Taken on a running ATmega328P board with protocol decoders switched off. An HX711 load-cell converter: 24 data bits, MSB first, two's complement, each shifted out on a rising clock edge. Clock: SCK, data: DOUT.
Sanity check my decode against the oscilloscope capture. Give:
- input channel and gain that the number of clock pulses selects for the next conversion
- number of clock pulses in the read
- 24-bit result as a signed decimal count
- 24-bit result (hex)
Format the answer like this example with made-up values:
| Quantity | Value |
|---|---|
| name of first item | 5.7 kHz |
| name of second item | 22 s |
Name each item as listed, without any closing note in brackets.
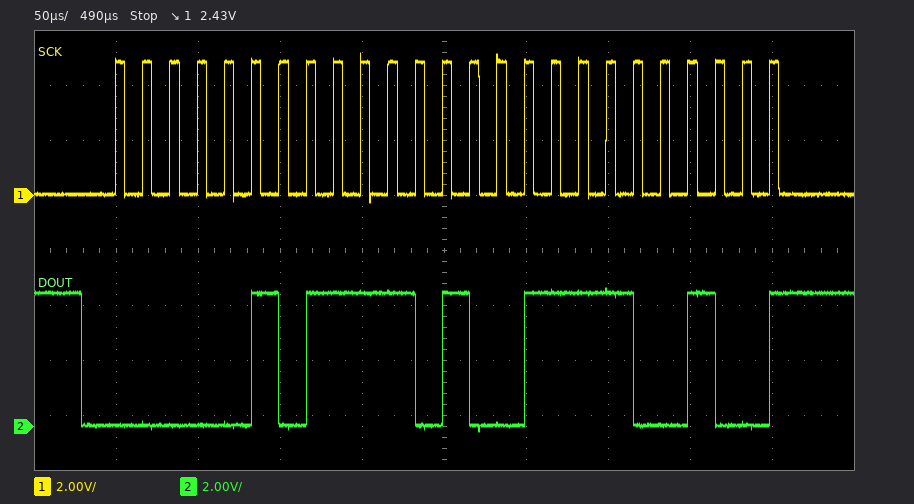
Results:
| Quantity | Value |
|---|---|
| input channel and gain that the number of clock pulses selects for the next conversion | channel A, gain 128 |
| number of clock pulses in the read | 25 |
| 24-bit result as a signed decimal count | 387556 |
| 24-bit result | 0x05E9E4 |
